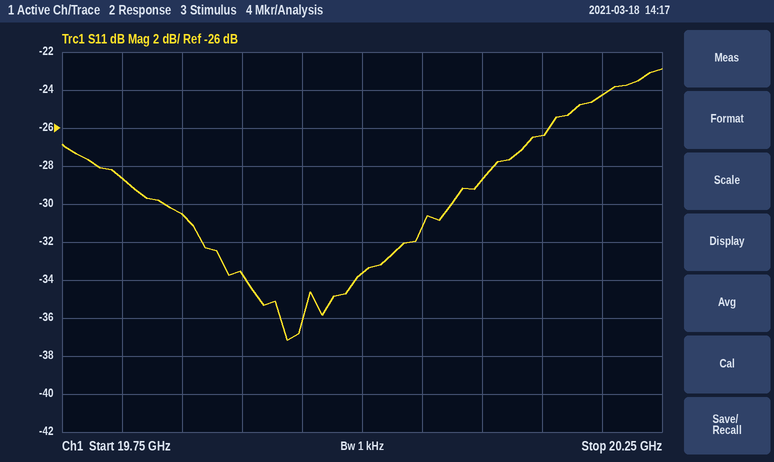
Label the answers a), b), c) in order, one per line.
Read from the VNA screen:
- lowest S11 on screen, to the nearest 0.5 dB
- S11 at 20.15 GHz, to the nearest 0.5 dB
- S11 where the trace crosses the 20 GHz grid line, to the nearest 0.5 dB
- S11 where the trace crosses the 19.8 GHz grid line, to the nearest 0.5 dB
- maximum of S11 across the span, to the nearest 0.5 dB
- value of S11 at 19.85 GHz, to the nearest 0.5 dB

a) -37.0 dB
b) -26.5 dB
c) -33.5 dB
d) -28.5 dB
e) -23.0 dB
f) -30.5 dB
